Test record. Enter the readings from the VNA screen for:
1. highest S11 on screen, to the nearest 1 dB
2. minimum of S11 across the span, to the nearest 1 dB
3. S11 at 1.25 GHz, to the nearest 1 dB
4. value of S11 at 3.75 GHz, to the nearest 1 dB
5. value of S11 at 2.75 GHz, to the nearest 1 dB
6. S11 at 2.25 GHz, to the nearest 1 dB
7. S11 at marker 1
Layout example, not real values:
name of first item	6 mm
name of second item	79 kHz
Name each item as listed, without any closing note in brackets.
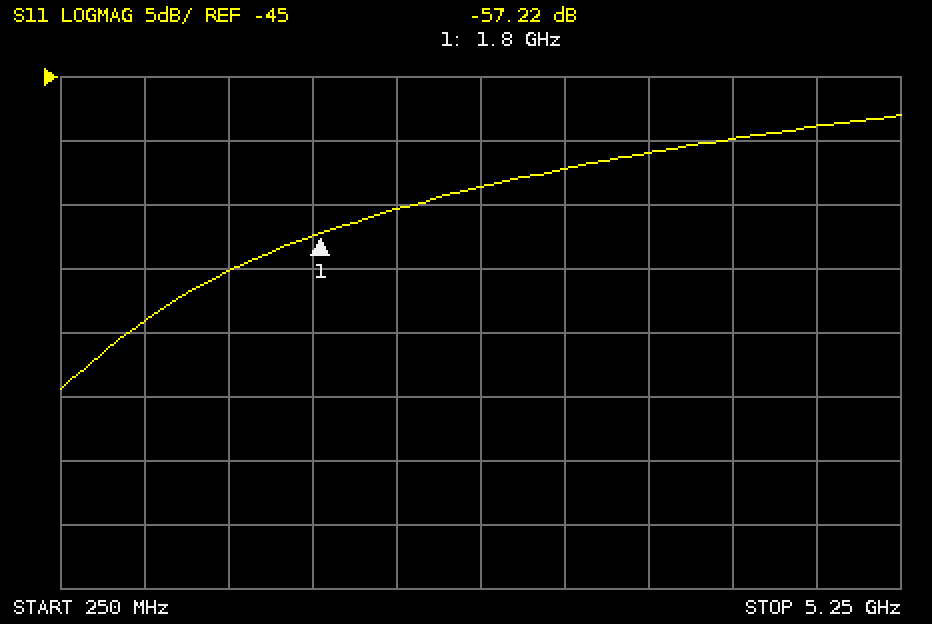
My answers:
highest S11 on screen, to the nearest 1 dB	-48 dB
minimum of S11 across the span, to the nearest 1 dB	-69 dB
S11 at 1.25 GHz, to the nearest 1 dB	-60 dB
value of S11 at 3.75 GHz, to the nearest 1 dB	-51 dB
value of S11 at 2.75 GHz, to the nearest 1 dB	-54 dB
S11 at 2.25 GHz, to the nearest 1 dB	-55 dB
S11 at marker 1	-57.22 dB
